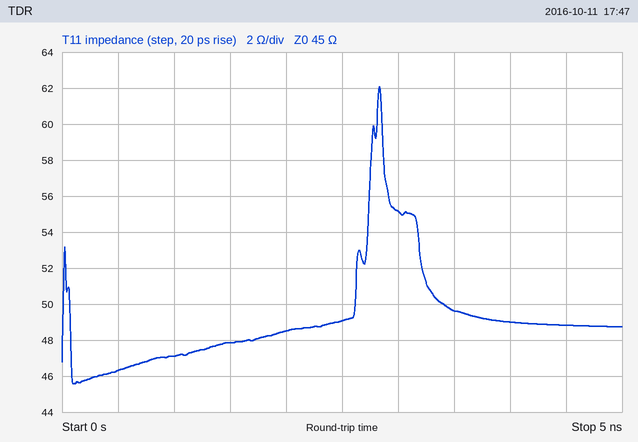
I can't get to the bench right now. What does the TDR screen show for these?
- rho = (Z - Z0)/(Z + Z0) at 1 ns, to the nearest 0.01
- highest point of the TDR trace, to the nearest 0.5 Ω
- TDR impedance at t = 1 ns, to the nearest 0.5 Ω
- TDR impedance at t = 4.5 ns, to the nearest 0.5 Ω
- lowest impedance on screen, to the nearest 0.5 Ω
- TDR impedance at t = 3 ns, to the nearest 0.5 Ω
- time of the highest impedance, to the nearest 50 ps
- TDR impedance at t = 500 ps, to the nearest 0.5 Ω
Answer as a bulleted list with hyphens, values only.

- +0.02
- 62.0 Ω
- 47.0 Ω
- 49.0 Ω
- 45.5 Ω
- 55.0 Ω
- 2.85 ns
- 46.5 Ω
